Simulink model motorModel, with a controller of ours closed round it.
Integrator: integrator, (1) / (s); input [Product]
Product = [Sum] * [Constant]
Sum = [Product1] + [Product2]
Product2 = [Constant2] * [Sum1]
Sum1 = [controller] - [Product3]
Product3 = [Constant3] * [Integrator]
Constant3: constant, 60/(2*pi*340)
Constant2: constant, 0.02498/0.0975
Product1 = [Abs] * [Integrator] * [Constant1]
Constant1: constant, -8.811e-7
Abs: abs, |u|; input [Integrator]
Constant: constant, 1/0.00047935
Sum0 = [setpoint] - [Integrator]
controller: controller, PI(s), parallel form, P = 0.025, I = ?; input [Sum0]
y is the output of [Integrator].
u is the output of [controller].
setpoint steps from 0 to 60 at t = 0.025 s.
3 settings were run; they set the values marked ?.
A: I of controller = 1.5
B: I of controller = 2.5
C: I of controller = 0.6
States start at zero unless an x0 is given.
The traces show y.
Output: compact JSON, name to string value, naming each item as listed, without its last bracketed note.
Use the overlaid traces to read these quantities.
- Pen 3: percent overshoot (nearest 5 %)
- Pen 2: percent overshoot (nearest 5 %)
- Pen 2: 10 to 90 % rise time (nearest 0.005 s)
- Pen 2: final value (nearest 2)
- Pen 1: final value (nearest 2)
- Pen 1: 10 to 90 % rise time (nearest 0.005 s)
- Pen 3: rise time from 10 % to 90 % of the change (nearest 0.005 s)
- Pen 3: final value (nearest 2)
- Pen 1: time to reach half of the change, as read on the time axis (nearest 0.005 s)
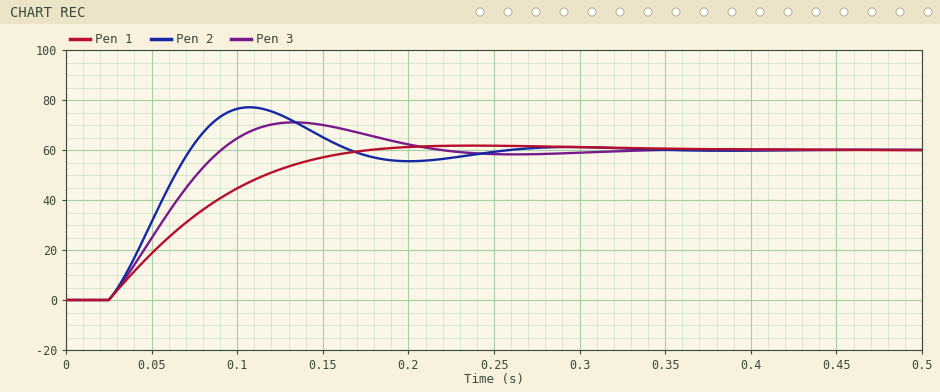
{"Pen 3: percent overshoot": "20 %", "Pen 2: percent overshoot": "30 %", "Pen 2: 10 to 90 % rise time": "0.035 s", "Pen 2: final value": "60", "Pen 1: final value": "60", "Pen 1: 10 to 90 % rise time": "0.100 s", "Pen 3: rise time from 10 % to 90 % of the change": "0.050 s", "Pen 3: final value": "60", "Pen 1: time to reach half of the change, as read on the time axis": "0.070 s"}
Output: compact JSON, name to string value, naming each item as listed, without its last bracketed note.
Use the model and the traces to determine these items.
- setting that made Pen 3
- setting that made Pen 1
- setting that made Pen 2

{"setting that made Pen 3": "A", "setting that made Pen 1": "C", "setting that made Pen 2": "B"}
